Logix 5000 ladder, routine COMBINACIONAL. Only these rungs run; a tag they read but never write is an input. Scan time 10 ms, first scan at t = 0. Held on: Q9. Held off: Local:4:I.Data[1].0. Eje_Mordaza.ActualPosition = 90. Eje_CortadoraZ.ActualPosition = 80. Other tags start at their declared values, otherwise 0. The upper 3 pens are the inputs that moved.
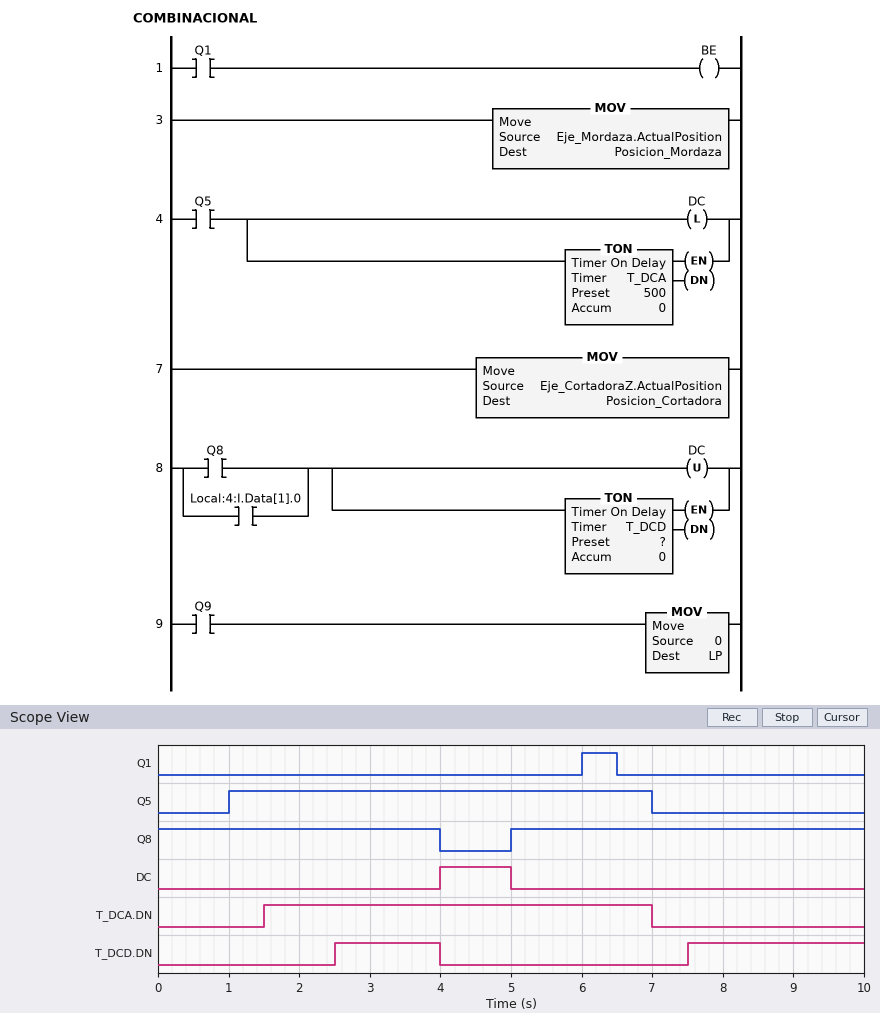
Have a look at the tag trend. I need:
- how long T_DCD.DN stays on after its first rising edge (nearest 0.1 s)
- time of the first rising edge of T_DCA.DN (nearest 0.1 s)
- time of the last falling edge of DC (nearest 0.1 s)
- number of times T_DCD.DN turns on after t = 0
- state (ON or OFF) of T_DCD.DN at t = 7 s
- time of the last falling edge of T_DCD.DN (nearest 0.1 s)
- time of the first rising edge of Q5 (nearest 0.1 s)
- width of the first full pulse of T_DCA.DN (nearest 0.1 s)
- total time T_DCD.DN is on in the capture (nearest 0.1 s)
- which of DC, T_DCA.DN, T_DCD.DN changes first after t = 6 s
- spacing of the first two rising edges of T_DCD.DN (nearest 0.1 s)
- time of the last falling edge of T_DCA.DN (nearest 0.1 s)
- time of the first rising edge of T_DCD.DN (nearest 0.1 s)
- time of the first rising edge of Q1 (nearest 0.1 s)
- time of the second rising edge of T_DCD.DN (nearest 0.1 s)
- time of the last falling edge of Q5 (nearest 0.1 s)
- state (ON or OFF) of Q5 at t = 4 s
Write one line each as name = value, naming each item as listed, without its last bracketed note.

how long T_DCD.DN stays on after its first rising edge = 1.5 s
time of the first rising edge of T_DCA.DN = 1.5 s
time of the last falling edge of DC = 5.0 s
number of times T_DCD.DN turns on after t = 0 = 2
state (ON or OFF) of T_DCD.DN at t = 7 s = OFF
time of the last falling edge of T_DCD.DN = 4.0 s
time of the first rising edge of Q5 = 1.0 s
width of the first full pulse of T_DCA.DN = 5.5 s
total time T_DCD.DN is on in the capture = 4.0 s
which of DC, T_DCA.DN, T_DCD.DN changes first after t = 6 s = T_DCA.DN
spacing of the first two rising edges of T_DCD.DN = 5.0 s
time of the last falling edge of T_DCA.DN = 7.0 s
time of the first rising edge of T_DCD.DN = 2.5 s
time of the first rising edge of Q1 = 6.0 s
time of the second rising edge of T_DCD.DN = 7.5 s
time of the last falling edge of Q5 = 7.0 s
state (ON or OFF) of Q5 at t = 4 s = ON
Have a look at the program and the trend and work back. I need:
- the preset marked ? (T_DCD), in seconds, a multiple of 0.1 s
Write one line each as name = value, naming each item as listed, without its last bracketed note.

the preset marked ? (T_DCD), in seconds, a multiple of 0.1 s = 2.5 s
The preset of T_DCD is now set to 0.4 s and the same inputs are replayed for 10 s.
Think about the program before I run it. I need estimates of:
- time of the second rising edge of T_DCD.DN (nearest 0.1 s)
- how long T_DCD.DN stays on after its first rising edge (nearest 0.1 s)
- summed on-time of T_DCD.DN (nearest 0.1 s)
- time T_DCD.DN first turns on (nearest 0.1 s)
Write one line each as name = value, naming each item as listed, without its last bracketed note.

time of the second rising edge of T_DCD.DN = 5.4 s
how long T_DCD.DN stays on after its first rising edge = 3.6 s
summed on-time of T_DCD.DN = 8.2 s
time T_DCD.DN first turns on = 0.4 s
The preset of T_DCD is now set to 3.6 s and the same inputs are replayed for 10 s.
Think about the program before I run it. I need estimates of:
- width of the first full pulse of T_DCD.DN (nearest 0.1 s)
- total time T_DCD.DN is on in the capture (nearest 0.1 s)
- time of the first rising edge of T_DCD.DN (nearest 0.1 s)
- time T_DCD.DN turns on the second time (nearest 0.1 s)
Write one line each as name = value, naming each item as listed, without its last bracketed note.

width of the first full pulse of T_DCD.DN = 0.4 s
total time T_DCD.DN is on in the capture = 1.8 s
time of the first rising edge of T_DCD.DN = 3.6 s
time T_DCD.DN turns on the second time = 8.6 s
